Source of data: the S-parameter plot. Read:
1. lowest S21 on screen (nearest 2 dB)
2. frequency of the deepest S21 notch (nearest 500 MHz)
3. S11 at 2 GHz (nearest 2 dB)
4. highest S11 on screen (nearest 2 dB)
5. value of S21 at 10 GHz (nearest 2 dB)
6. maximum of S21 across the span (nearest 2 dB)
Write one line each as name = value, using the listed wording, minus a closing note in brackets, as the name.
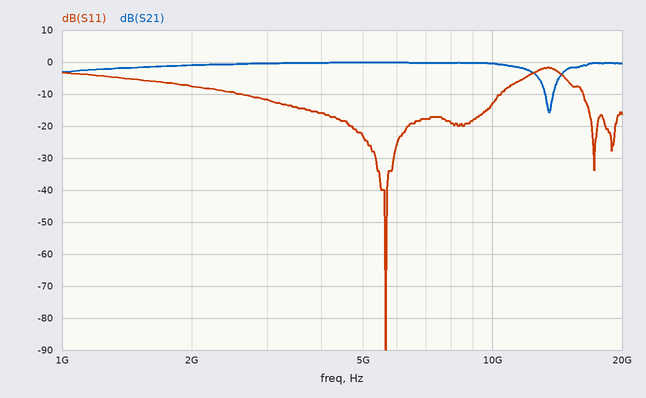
lowest S21 on screen = -16 dB
frequency of the deepest S21 notch = 13.5 GHz
S11 at 2 GHz = -8 dB
highest S11 on screen = -2 dB
value of S21 at 10 GHz = 0 dB
maximum of S21 across the span = 0 dB
